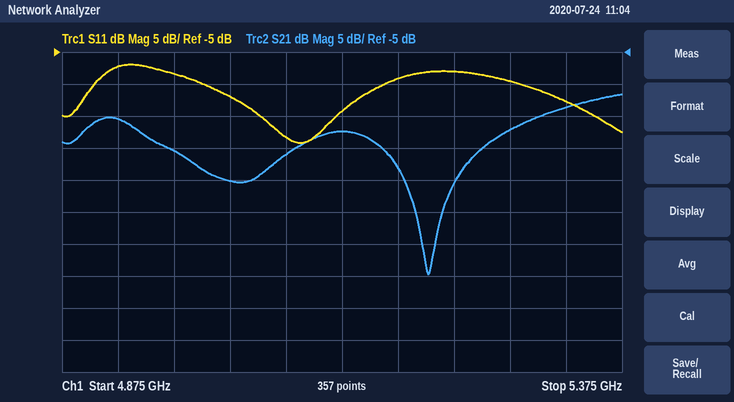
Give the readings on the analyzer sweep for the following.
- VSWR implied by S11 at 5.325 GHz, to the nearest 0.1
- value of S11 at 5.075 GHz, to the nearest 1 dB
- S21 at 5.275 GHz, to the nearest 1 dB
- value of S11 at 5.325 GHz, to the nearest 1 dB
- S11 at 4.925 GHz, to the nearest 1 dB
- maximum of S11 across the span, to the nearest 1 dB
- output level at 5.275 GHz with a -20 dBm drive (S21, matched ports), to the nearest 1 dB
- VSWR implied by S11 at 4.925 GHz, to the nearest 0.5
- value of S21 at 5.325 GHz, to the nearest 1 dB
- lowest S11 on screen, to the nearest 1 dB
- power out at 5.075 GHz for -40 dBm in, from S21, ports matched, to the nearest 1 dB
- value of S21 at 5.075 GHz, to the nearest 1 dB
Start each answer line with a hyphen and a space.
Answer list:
- 1.6
- -18 dB
- -17 dB
- -13 dB
- -7 dB
- -7 dB
- -37 dBm
- 2.5
- -14 dB
- -19 dB
- -61 dBm
- -21 dB
